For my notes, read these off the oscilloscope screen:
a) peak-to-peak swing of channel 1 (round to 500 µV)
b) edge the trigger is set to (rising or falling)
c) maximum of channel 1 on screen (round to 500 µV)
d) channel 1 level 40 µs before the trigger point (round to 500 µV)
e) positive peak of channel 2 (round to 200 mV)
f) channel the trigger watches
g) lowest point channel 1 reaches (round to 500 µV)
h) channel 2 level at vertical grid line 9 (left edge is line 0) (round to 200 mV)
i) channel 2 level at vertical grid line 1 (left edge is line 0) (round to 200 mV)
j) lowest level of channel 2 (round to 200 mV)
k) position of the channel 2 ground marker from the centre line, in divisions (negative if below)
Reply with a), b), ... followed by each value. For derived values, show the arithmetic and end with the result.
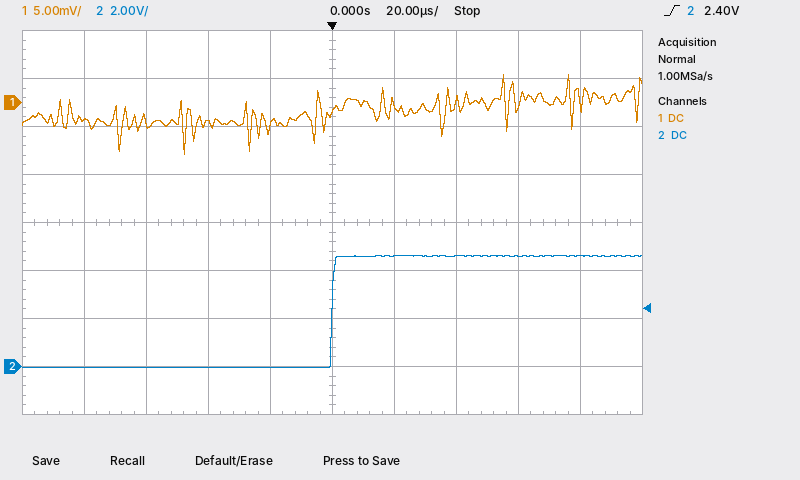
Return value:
a) 3.0 mV − (-5.5 mV) = 8.5 mV
b) rising
c) 3.0 mV
d) -2.0 mV
e) 4.6 V
f) channel 2
g) -5.5 mV
h) 4.6 V
i) 0.0 V
j) 0.0 V
k) -3.0 div
